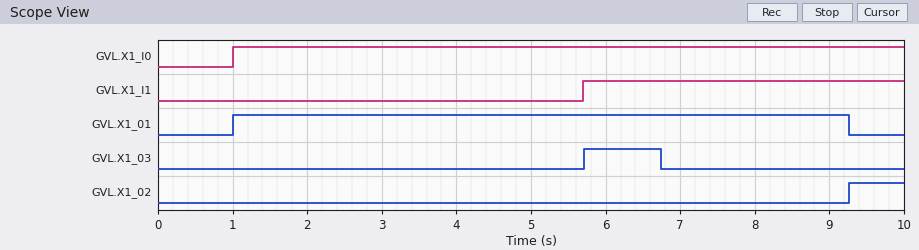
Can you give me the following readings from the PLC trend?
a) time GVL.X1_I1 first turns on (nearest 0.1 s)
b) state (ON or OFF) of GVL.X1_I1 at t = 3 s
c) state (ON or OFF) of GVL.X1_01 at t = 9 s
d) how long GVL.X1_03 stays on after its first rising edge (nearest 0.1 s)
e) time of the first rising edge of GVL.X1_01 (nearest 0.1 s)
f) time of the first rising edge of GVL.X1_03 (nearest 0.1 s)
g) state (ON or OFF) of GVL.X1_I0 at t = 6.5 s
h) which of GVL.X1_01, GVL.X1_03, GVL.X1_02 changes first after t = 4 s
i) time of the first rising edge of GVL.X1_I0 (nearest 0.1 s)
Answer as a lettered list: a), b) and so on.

a) 5.7 s
b) OFF
c) ON
d) 1.0 s
e) 1.0 s
f) 5.7 s
g) ON
h) GVL.X1_03
i) 1.0 s
